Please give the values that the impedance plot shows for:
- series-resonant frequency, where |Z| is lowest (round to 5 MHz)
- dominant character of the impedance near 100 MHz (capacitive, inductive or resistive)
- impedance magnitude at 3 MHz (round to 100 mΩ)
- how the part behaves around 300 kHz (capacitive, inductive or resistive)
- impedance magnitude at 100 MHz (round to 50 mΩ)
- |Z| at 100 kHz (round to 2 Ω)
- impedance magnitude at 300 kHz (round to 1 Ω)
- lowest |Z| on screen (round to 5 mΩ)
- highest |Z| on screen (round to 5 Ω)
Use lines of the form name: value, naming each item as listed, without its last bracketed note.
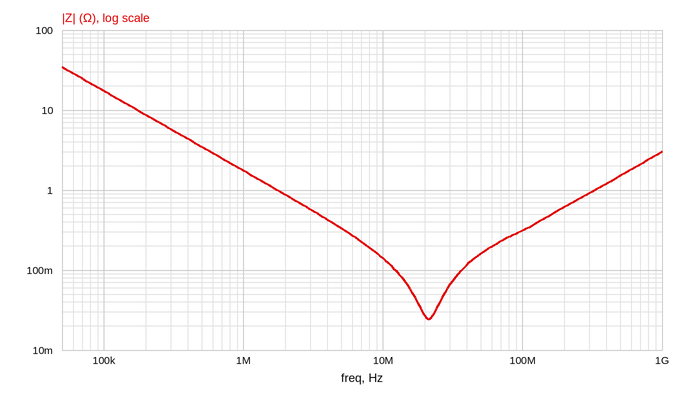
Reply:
series-resonant frequency, where |Z| is lowest: 20 MHz
dominant character of the impedance near 100 MHz: inductive
impedance magnitude at 3 MHz: 600 mΩ
how the part behaves around 300 kHz: capacitive
impedance magnitude at 100 MHz: 300 mΩ
|Z| at 100 kHz: 18 Ω
impedance magnitude at 300 kHz: 6 Ω
lowest |Z| on screen: 25 mΩ
highest |Z| on screen: 35 Ω
